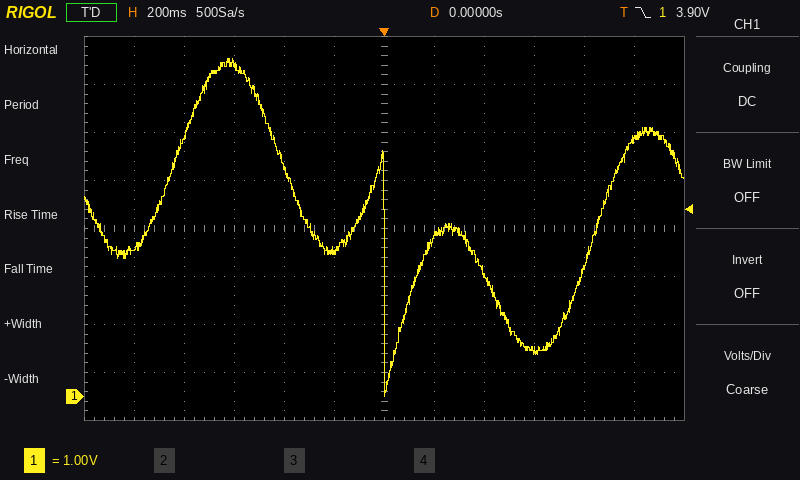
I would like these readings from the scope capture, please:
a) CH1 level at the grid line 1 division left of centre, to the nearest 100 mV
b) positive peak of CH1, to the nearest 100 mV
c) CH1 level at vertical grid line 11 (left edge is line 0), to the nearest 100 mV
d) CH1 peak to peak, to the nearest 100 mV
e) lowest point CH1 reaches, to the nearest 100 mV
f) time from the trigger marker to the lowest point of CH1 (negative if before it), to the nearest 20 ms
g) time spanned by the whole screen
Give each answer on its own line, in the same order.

3.0 V
7.0 V
5.4 V
7.0 V
0.0 V
0 ms
2.4 s
